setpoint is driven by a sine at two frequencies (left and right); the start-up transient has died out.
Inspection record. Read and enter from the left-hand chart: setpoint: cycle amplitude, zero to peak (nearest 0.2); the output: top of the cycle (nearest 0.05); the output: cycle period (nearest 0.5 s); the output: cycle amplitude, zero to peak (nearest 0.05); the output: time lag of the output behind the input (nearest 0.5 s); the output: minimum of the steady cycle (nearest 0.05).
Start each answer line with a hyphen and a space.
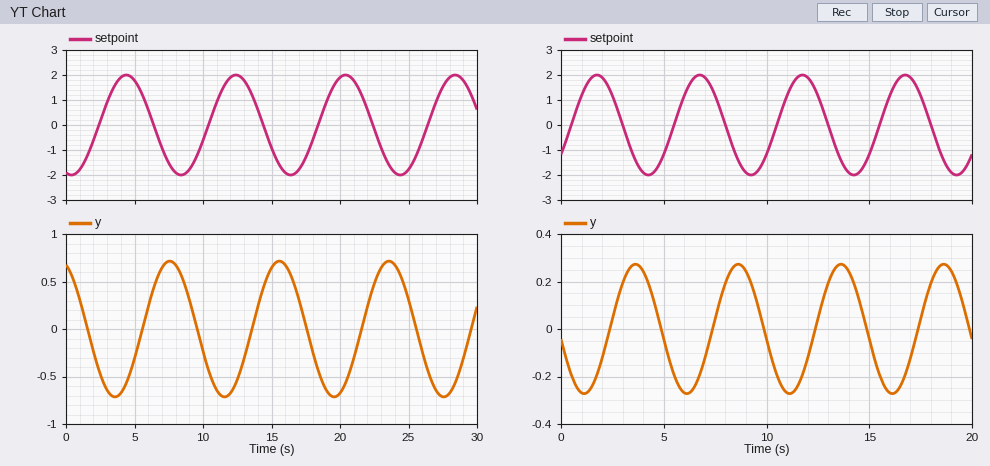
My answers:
- 2.0
- 0.70
- 8.0 s
- 0.70
- 3.0 s
- -0.70
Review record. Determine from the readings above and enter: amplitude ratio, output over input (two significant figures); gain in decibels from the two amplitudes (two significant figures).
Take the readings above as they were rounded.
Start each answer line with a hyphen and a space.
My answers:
- 0.35
- -9.1 dB
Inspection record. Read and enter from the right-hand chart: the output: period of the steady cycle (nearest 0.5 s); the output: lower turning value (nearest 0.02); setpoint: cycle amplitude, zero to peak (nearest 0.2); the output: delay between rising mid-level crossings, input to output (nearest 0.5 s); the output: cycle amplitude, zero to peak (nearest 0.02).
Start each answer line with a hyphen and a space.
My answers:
- 5.0 s
- -0.28
- 2.0
- 2.0 s
- 0.28
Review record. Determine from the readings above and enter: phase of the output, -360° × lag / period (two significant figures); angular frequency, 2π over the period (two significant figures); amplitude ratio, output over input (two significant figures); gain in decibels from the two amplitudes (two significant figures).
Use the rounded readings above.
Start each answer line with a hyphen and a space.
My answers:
- -140°
- 1.3 rad/s
- 0.14
- -17 dB
